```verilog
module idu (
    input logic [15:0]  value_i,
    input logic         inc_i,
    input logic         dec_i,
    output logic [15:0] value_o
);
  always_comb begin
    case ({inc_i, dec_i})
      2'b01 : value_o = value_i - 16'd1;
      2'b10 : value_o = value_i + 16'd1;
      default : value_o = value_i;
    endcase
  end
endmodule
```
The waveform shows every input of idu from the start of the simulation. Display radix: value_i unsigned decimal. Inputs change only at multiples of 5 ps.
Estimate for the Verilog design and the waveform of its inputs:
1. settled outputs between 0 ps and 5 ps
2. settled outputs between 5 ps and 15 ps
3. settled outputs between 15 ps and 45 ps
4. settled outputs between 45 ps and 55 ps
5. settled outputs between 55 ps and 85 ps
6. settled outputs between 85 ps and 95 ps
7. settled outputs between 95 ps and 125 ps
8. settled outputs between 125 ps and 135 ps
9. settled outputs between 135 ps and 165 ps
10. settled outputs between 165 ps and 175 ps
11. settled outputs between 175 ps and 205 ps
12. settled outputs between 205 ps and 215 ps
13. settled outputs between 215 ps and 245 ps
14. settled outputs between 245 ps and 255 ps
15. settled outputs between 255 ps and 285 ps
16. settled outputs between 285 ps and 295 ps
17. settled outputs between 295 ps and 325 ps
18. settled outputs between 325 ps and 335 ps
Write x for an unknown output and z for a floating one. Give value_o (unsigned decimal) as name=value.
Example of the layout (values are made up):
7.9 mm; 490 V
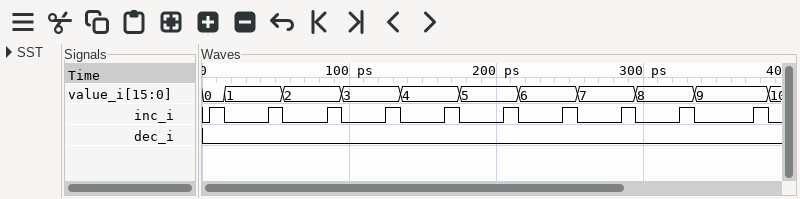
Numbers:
value_o=0; value_o=1; value_o=1; value_o=2; value_o=2; value_o=3; value_o=3; value_o=4; value_o=4; value_o=5; value_o=5; value_o=6; value_o=6; value_o=7; value_o=7; value_o=8; value_o=8; value_o=9
